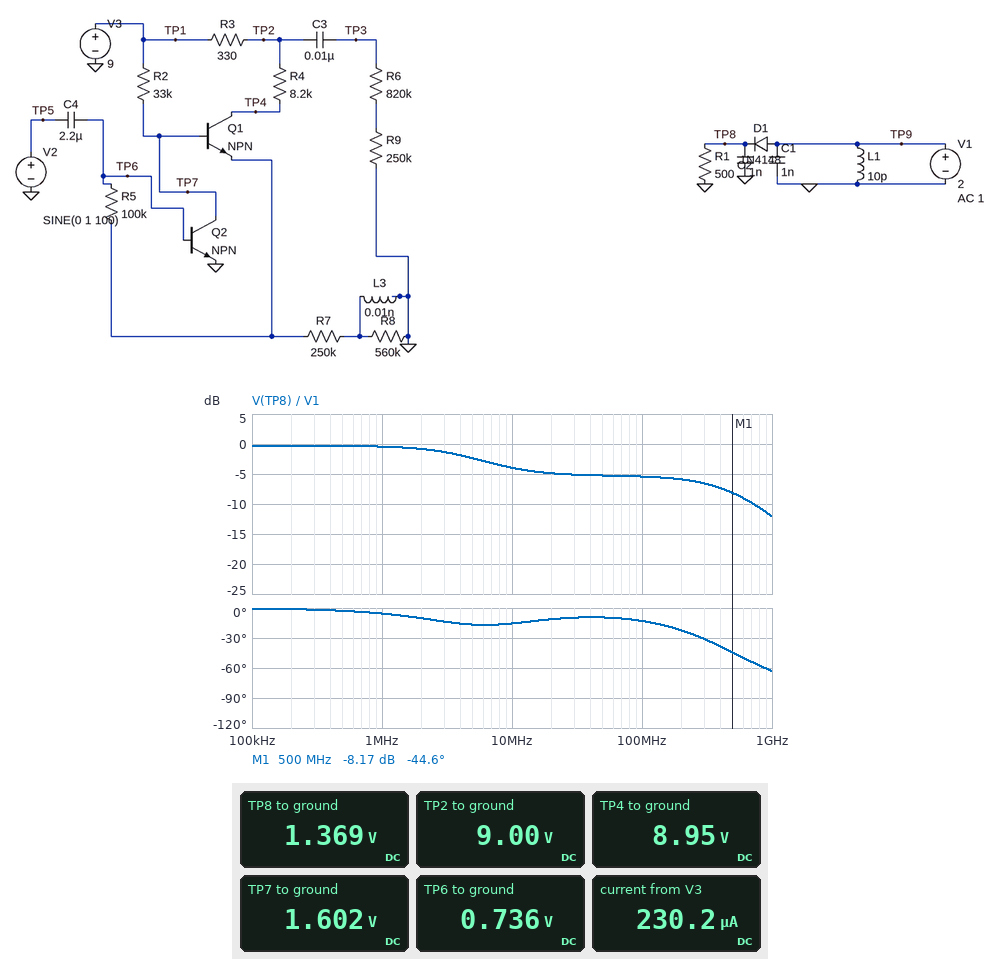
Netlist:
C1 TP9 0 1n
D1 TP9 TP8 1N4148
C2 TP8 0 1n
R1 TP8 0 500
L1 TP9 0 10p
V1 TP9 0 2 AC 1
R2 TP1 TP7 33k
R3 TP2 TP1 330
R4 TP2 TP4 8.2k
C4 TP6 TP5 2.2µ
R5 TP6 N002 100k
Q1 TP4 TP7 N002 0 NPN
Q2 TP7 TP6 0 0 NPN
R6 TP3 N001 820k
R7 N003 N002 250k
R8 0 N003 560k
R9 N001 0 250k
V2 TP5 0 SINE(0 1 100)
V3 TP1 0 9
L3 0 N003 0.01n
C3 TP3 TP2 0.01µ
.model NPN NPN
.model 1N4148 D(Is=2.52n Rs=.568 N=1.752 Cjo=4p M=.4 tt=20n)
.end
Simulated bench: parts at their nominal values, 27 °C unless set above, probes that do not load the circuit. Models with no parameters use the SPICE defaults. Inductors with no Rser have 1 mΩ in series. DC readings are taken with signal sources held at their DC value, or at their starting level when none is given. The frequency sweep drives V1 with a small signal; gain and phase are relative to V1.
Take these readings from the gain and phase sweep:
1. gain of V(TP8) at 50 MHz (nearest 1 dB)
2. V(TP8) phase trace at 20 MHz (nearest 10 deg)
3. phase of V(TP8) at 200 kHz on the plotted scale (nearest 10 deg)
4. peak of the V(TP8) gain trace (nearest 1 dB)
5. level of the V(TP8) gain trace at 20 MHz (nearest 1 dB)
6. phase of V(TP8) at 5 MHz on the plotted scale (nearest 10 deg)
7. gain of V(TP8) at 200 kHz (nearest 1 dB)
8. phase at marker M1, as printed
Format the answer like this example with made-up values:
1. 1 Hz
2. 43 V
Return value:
1. -5 dB
2. -10 deg
3. 0 deg
4. 0 dB
5. -5 dB
6. -20 deg
7. 0 dB
8. -44.6 deg
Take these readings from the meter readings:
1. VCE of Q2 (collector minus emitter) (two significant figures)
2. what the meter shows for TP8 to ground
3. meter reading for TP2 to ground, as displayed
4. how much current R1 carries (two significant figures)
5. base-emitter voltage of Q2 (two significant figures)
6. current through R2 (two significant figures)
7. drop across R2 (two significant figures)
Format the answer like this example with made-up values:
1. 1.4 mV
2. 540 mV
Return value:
1. 1.6 V
2. 1.369 V
3. 9.00 V
4. 2.7 mA
5. 740 mV
6. 220 µA
7. 7.4 V
